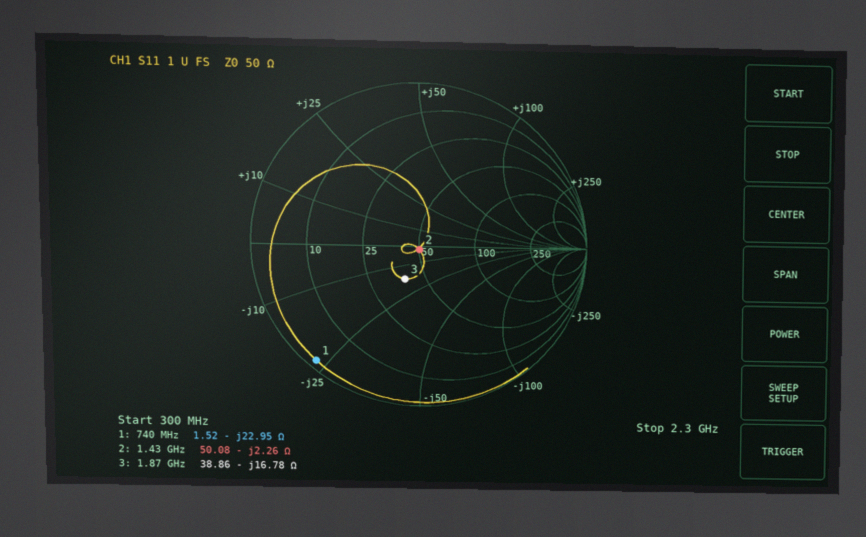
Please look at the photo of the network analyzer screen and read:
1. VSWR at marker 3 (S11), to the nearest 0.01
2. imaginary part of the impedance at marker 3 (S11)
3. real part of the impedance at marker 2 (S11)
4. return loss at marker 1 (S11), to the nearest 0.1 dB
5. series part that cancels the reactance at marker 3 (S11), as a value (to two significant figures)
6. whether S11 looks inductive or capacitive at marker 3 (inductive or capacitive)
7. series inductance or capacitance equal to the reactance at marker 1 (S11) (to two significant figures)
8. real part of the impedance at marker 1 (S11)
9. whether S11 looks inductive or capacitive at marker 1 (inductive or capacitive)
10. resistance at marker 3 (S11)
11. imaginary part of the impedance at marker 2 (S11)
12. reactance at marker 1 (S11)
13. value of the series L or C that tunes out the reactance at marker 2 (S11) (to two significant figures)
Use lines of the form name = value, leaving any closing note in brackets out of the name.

VSWR at marker 3 (S11), to the nearest 0.01 = 1.57
imaginary part of the impedance at marker 3 = -16.78 Ω
real part of the impedance at marker 2 = 50.08 Ω
return loss at marker 1 (S11), to the nearest 0.1 dB = 0.4 dB
series part that cancels the reactance at marker 3 (S11), as a value = 1.4 nH
whether S11 looks inductive or capacitive at marker 3 = capacitive
series inductance or capacitance equal to the reactance at marker 1 (S11) = 9.4 pF
real part of the impedance at marker 1 = 1.52 Ω
whether S11 looks inductive or capacitive at marker 1 = capacitive
resistance at marker 3 = 38.86 Ω
imaginary part of the impedance at marker 2 = -2.26 Ω
reactance at marker 1 = -22.95 Ω
value of the series L or C that tunes out the reactance at marker 2 (S11) = 250 pH
